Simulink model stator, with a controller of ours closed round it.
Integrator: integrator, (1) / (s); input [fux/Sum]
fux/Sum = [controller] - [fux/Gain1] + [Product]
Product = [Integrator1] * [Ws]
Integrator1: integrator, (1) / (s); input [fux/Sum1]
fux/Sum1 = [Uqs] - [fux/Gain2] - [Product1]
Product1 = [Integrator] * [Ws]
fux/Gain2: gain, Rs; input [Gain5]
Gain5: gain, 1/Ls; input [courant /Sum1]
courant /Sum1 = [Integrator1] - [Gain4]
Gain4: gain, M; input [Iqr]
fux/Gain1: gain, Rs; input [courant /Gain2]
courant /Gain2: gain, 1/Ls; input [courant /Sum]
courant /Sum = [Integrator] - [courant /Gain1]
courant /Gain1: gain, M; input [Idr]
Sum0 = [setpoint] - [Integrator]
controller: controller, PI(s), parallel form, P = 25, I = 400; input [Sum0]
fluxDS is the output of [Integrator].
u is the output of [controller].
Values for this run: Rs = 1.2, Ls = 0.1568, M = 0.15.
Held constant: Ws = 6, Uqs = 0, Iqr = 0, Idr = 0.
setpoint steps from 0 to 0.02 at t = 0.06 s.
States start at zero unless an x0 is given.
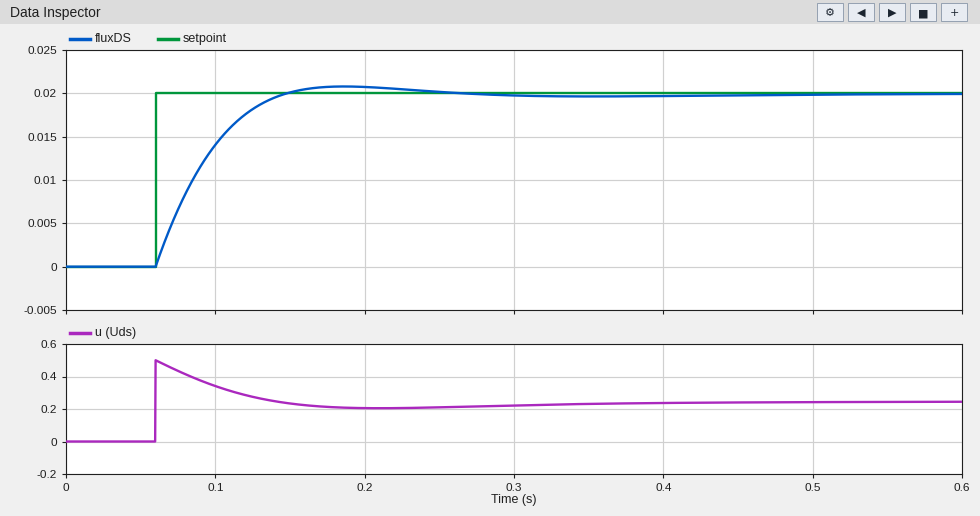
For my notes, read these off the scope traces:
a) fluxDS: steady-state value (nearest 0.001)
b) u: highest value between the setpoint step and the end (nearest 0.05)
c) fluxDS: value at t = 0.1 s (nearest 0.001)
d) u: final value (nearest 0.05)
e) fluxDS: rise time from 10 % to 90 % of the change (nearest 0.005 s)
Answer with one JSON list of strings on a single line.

["0.020", "0.50", "0.014", "0.25", "0.060 s"]
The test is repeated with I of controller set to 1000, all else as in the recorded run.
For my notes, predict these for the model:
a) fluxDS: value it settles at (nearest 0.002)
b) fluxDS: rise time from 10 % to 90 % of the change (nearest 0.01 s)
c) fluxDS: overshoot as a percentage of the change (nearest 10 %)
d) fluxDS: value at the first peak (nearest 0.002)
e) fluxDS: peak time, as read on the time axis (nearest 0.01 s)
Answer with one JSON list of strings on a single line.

["0.020", "0.04 s", "20 %", "0.024", "0.14 s"]
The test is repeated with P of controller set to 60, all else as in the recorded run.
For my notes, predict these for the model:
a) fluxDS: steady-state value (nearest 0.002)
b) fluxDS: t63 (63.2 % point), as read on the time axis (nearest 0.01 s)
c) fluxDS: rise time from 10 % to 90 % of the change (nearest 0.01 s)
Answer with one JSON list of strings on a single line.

["0.020", "0.08 s", "0.04 s"]
